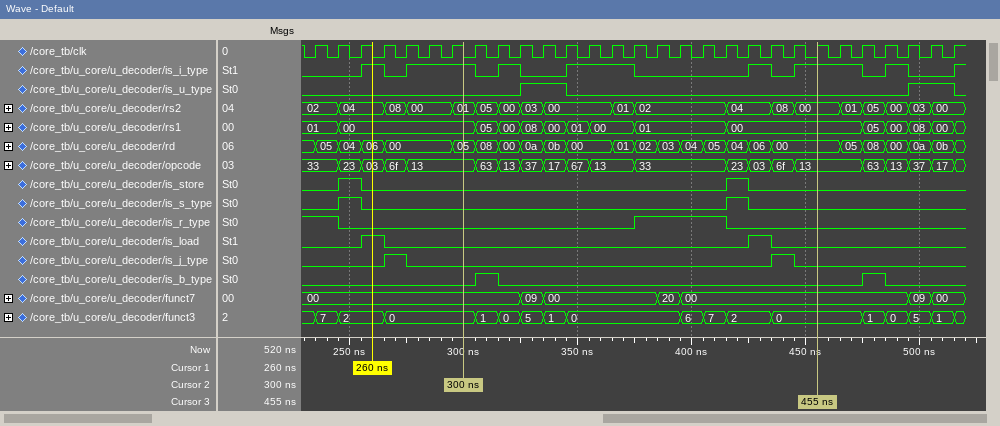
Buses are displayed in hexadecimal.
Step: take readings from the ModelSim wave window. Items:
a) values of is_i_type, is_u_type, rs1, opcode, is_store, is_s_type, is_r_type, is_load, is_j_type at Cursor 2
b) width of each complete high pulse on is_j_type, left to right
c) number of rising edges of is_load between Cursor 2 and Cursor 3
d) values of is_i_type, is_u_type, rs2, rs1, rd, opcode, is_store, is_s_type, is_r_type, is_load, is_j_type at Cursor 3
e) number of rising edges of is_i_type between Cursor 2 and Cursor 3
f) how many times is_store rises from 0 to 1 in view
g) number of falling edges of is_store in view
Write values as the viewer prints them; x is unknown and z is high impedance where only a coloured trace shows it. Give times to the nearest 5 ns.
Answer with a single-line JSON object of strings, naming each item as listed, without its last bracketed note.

{"values of is_i_type, is_u_type, rs1, opcode, is_store, is_s_type, is_r_type, is_load, is_j_type at Cursor 2": "is_i_type=1, is_u_type=0, rs1=00, opcode=13, is_store=0, is_s_type=0, is_r_type=0, is_load=0, is_j_type=0", "width of each complete high pulse on is_j_type, left to right": "10 ns, 10 ns", "number of rising edges of is_load between Cursor 2 and Cursor 3": "1", "values of is_i_type, is_u_type, rs2, rs1, rd, opcode, is_store, is_s_type, is_r_type, is_load, is_j_type at Cursor 3": "is_i_type=1, is_u_type=0, rs2=00, rs1=00, rd=00, opcode=13, is_store=0, is_s_type=0, is_r_type=0, is_load=0, is_j_type=0", "number of rising edges of is_i_type between Cursor 2 and Cursor 3": "4", "how many times is_store rises from 0 to 1 in view": "2", "number of falling edges of is_store in view": "2"}
